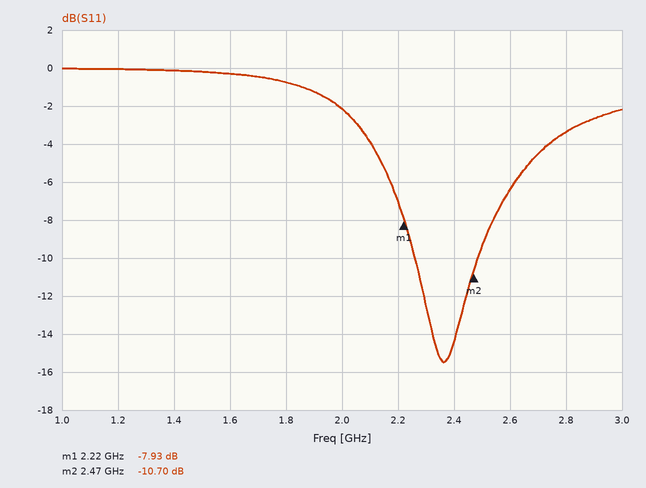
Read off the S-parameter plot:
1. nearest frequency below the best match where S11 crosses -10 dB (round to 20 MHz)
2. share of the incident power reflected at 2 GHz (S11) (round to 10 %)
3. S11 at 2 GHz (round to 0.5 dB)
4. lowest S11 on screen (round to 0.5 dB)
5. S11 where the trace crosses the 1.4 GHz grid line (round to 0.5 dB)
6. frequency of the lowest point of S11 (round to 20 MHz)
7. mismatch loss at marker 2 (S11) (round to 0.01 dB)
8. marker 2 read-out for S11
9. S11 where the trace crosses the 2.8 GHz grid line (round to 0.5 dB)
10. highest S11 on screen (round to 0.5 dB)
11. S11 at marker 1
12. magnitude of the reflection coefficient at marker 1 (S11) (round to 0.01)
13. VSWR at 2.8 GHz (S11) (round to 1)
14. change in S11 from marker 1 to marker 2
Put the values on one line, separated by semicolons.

2.26 GHz; 60 %; -2.0 dB; -15.5 dB; 0.0 dB; 2.36 GHz; 0.39 dB; -10.70 dB; -3.5 dB; 0.0 dB; -7.93 dB; 0.40; 5; -2.77 dB
